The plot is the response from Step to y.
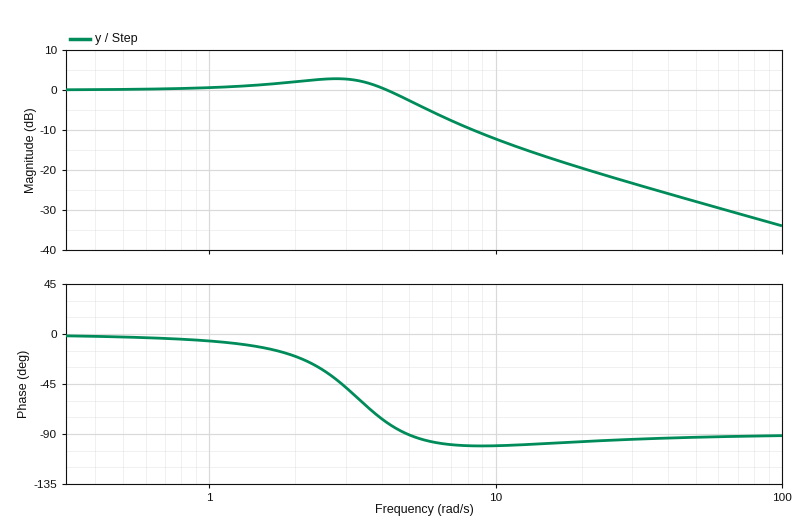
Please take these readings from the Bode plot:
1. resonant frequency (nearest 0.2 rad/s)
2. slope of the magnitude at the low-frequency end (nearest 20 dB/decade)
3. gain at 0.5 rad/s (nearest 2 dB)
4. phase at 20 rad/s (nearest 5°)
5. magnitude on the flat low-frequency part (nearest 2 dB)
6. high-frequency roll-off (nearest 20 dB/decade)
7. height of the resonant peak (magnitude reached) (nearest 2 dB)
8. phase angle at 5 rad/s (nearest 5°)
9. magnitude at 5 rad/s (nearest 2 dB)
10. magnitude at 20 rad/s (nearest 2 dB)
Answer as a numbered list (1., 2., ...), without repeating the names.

1. 2.8 rad/s
2. 0 dB/decade
3. 0 dB
4. -95°
5. 0 dB
6. -20 dB/decade
7. 2 dB
8. -90°
9. -2 dB
10. -20 dB
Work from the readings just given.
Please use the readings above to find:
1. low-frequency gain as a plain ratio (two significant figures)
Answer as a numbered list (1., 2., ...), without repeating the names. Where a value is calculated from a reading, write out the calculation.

1. 10^(0 / 20) = 1.0
